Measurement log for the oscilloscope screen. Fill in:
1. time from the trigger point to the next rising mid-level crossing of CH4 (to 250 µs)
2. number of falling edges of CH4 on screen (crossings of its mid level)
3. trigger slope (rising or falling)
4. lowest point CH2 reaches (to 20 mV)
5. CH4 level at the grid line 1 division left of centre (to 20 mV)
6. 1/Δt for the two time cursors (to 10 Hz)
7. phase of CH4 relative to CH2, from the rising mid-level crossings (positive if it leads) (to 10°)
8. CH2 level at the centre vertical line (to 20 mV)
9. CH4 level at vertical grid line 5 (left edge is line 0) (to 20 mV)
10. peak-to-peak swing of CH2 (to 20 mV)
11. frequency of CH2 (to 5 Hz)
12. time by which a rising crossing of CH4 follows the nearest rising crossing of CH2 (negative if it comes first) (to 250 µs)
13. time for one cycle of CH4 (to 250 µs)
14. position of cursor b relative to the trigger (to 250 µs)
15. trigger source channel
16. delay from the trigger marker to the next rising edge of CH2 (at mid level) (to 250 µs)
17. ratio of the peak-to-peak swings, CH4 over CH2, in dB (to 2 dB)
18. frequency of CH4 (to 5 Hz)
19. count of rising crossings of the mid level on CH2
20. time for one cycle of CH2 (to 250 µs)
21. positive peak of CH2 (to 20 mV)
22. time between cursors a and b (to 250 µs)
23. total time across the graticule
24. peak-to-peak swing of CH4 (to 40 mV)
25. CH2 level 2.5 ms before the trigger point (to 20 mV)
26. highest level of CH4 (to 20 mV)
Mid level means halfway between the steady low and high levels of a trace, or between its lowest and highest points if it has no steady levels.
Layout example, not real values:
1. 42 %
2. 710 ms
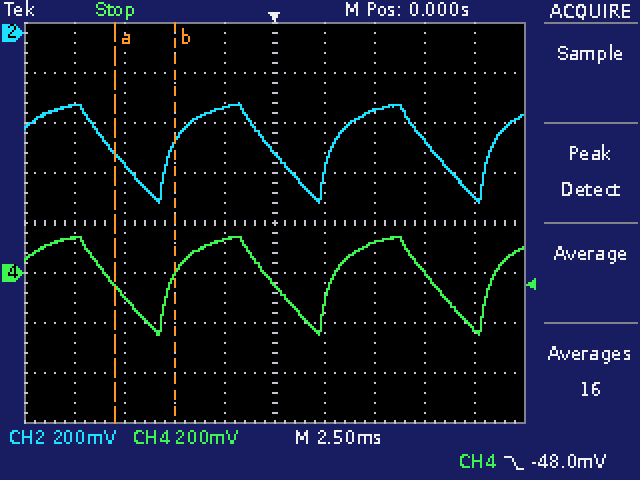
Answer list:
1. 2.75 ms
2. 3
3. falling
4. -680 mV
5. 140 mV
6. 330 Hz
7. 0°
8. -480 mV
9. -40 mV
10. 400 mV
11. 125 Hz
12. 0.00 ms
13. 8.00 ms
14. -5.00 ms
15. CH4
16. 2.75 ms
17. 0 dB
18. 125 Hz
19. 3
20. 8.00 ms
21. -280 mV
22. 3.00 ms
23. 25 ms
24. 400 mV
25. -300 mV
26. 140 mV
